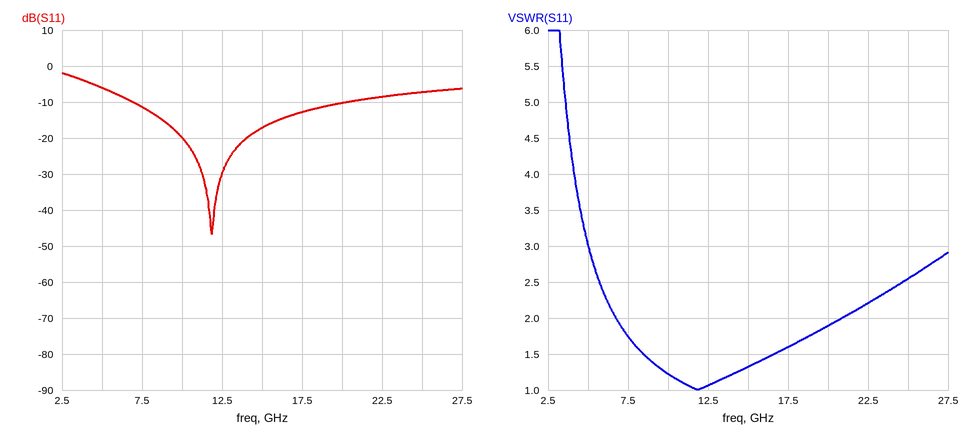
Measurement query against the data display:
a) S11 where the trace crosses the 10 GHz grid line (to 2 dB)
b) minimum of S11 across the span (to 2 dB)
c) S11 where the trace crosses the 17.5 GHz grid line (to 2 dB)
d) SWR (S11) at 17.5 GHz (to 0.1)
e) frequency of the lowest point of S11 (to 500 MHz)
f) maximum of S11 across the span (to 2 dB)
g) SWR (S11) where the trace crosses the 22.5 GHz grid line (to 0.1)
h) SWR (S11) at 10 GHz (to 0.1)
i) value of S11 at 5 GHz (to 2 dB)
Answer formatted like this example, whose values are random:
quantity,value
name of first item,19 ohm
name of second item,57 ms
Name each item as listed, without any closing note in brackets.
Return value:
quantity,value
S11 where the trace crosses the 10 GHz grid line,-20 dB
minimum of S11 across the span,-46 dB
S11 where the trace crosses the 17.5 GHz grid line,-12 dB
SWR (S11) at 17.5 GHz,1.6
frequency of the lowest point of S11,12.0 GHz
maximum of S11 across the span,-2 dB
SWR (S11) where the trace crosses the 22.5 GHz grid line,2.2
SWR (S11) at 10 GHz,1.2
value of S11 at 5 GHz,-6 dB
